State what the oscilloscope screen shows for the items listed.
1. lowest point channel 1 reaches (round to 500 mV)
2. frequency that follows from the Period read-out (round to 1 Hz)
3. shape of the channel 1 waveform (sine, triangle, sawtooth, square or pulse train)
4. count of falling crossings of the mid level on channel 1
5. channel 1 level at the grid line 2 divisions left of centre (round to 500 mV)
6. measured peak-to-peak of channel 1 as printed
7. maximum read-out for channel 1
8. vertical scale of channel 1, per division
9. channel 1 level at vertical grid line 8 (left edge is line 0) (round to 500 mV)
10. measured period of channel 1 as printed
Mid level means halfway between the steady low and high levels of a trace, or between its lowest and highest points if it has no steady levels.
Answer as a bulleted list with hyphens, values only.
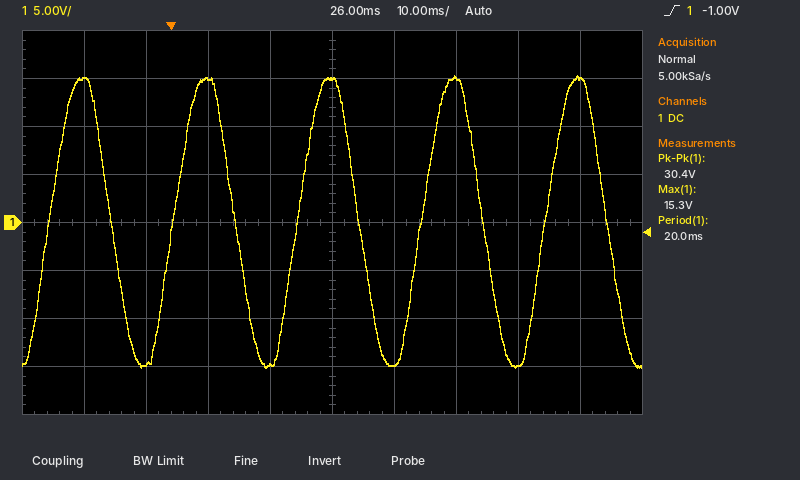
- -15.0 V
- 50 Hz
- sine
- 5
- 15.0 V
- 30.4 V
- 15.3 V
- 5 V
- -15.0 V
- 20.0 ms
